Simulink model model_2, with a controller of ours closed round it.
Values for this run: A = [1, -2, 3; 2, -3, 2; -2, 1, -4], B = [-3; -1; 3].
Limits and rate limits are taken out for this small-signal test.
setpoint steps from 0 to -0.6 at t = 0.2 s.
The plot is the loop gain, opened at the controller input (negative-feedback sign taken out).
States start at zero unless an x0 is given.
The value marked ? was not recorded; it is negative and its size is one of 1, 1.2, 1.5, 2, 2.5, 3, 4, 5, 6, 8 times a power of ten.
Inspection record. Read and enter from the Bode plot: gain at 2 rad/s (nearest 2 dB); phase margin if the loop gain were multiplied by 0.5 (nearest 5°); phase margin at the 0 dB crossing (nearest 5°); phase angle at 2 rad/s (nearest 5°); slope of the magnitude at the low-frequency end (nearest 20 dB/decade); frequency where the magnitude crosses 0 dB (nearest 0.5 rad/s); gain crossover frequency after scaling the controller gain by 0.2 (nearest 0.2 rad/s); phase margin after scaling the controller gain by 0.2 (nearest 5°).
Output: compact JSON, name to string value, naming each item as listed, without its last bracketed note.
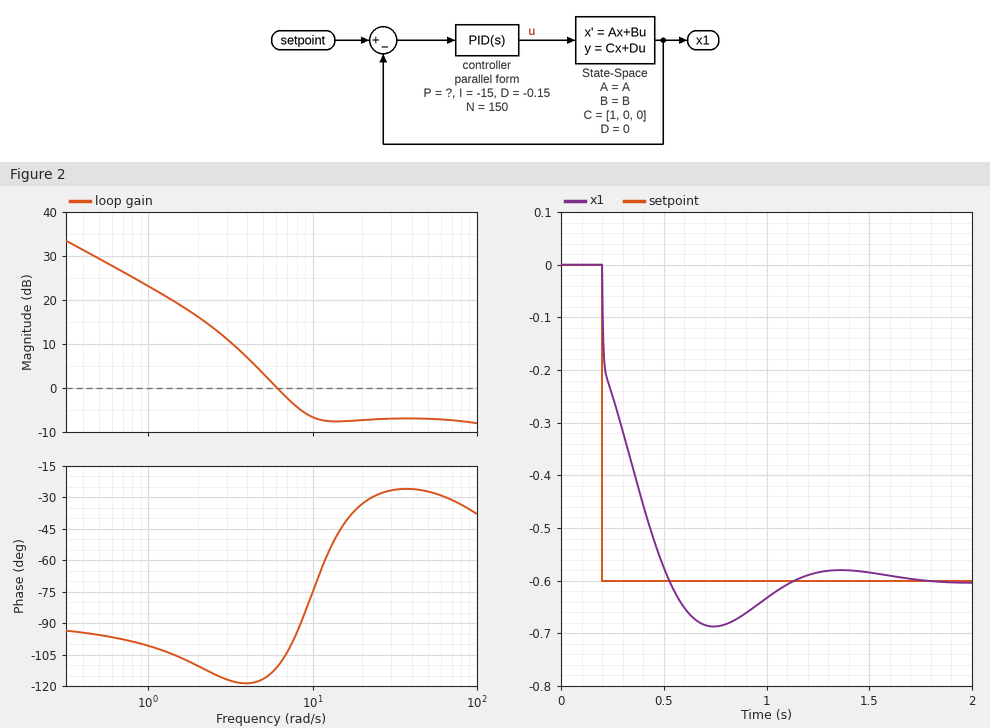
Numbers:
{"gain at 2 rad/s": "16 dB", "phase margin if the loop gain were multiplied by 0.5": "60°", "phase margin at the 0 dB crossing": "70°", "phase angle at 2 rad/s": "-110°", "slope of the magnitude at the low-frequency end": "-20 dB/decade", "frequency where the magnitude crosses 0 dB": "6.0 rad/s", "gain crossover frequency after scaling the controller gain by 0.2": "2.4 rad/s", "phase margin after scaling the controller gain by 0.2": "65°"}
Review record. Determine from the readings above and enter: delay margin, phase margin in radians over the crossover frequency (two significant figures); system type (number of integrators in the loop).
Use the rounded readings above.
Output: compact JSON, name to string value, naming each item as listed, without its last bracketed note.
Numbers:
{"delay margin, phase margin in radians over the crossover frequency": "0.20 s", "system type": "1"}
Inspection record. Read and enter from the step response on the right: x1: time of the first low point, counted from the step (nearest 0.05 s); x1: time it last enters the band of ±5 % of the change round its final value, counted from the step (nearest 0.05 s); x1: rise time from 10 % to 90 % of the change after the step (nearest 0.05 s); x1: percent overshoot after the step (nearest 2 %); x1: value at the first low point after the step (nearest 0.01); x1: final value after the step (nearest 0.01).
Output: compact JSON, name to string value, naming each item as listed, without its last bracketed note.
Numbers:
{"x1: time of the first low point, counted from the step": "0.55 s", "x1: time it last enters the band of ±5 % of the change round its final value, counted from the step": "0.80 s", "x1: rise time from 10 % to 90 % of the change after the step": "0.25 s", "x1: percent overshoot after the step": "14 %", "x1: value at the first low point after the step": "-0.69", "x1: final value after the step": "-0.60"}
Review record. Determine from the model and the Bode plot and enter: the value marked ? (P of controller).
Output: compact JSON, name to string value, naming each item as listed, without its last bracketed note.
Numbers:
{"the value marked ?": "-1.5"}
